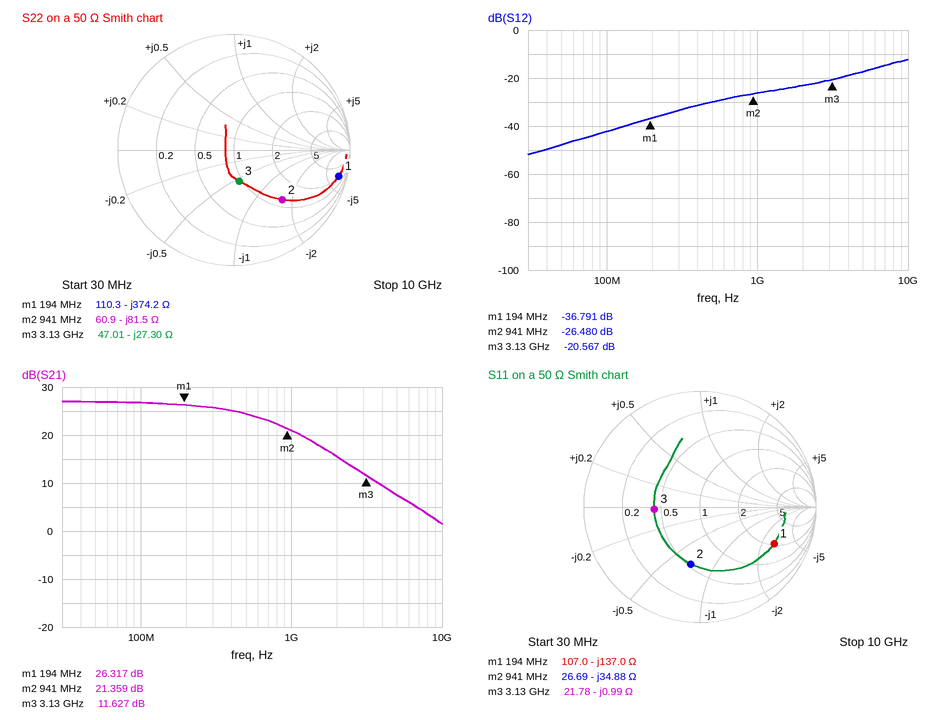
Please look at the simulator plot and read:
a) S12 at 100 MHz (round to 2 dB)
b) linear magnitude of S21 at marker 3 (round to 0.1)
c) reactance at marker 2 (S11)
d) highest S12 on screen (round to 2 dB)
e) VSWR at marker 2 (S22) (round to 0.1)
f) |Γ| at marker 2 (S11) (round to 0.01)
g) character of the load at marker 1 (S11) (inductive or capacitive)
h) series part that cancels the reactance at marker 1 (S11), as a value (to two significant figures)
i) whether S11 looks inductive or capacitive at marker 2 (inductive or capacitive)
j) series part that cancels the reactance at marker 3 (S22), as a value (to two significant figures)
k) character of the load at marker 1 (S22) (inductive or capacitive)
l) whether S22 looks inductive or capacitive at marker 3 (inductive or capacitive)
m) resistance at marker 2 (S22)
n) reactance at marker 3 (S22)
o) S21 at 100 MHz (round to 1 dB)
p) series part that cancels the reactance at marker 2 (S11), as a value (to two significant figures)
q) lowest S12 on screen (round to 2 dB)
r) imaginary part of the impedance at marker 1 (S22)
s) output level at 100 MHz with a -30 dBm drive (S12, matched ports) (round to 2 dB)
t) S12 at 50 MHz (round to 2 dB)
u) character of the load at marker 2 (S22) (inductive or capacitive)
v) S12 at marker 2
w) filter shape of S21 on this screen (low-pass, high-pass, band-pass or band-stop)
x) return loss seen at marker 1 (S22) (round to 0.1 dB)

-42 dB
3.8
-34.88 Ω
-12 dB
4.0
0.50
capacitive
110 nH
capacitive
1.4 nH
capacitive
capacitive
60.9 Ω
-27.30 Ω
27 dB
5.9 nH
-52 dB
-374.2 Ω
-72 dBm
-48 dB
capacitive
-26.480 dB
low-pass
0.6 dB
